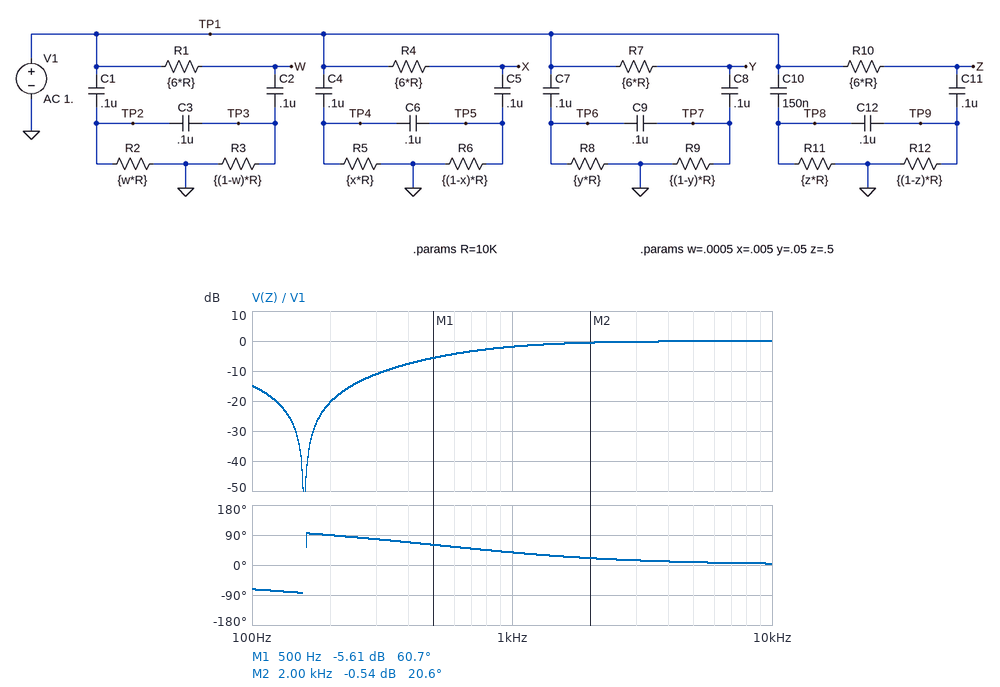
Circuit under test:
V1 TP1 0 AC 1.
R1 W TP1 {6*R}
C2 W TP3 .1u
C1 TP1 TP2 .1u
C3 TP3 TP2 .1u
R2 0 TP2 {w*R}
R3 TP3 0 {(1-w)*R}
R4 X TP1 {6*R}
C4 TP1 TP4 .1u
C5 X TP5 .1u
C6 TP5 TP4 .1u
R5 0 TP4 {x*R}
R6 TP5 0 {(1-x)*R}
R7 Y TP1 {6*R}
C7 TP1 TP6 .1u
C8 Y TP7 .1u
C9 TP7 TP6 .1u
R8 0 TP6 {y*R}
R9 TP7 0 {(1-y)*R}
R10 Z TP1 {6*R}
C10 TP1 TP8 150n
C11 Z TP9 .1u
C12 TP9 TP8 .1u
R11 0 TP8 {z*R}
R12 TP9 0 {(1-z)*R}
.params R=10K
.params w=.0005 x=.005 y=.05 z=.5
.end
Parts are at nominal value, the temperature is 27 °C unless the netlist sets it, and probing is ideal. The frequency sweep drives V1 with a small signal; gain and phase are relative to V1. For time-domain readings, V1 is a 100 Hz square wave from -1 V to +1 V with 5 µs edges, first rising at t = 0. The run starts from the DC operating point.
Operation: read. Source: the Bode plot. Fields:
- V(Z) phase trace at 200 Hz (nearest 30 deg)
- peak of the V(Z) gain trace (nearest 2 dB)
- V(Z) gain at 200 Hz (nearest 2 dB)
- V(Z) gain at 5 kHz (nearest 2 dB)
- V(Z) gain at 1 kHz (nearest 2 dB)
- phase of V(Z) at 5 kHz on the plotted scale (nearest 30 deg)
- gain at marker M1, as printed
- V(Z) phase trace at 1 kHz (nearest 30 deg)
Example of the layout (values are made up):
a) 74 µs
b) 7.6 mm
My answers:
a) 90 deg
b) 0 dB
c) -20 dB
d) 0 dB
e) -2 dB
f) 0 deg
g) -5.61 dB
h) 30 deg
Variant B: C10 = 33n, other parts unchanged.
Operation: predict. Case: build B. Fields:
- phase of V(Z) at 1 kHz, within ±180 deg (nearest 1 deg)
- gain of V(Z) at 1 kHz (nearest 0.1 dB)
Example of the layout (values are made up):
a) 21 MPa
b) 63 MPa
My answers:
a) 68 deg
b) -8.5 dB
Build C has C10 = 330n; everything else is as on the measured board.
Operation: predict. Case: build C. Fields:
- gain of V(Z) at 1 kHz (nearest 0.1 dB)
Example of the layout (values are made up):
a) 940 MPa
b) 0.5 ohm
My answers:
a) -1.0 dB
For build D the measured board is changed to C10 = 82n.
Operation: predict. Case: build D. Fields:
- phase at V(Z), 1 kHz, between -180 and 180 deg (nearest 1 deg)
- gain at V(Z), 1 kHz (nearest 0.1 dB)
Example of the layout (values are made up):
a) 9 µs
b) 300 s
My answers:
a) 50 deg
b) -3.5 dB
